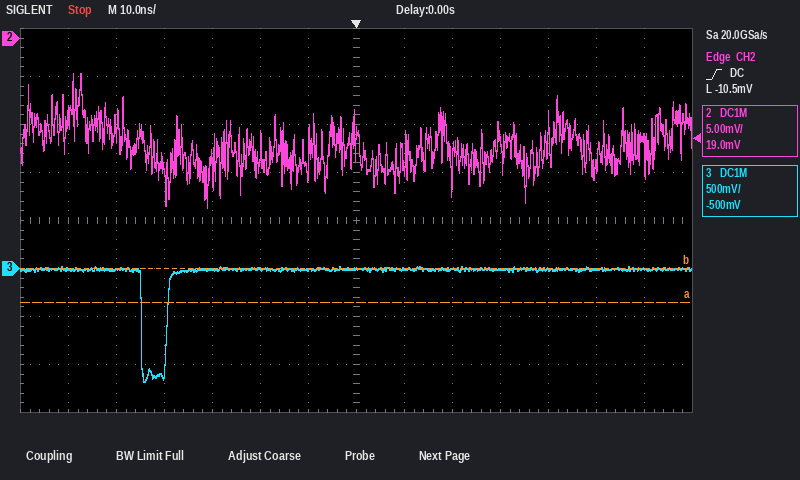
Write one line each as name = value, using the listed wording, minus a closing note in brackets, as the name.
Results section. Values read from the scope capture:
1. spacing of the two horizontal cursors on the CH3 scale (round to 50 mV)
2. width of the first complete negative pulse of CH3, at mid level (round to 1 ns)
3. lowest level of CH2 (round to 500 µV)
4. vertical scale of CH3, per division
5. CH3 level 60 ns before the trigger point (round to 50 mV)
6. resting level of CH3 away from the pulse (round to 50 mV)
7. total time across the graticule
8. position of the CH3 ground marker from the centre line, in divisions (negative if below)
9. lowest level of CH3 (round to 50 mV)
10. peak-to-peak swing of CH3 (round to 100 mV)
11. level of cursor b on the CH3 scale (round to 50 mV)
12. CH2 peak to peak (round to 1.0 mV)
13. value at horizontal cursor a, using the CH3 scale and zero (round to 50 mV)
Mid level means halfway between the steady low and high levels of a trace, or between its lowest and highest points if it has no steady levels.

spacing of the two horizontal cursors on the CH3 scale = 350 mV
width of the first complete negative pulse of CH3, at mid level = 5 ns
lowest level of CH2 = -17.5 mV
vertical scale of CH3, per division = 500 mV
CH3 level 60 ns before the trigger point = 0 mV
resting level of CH3 away from the pulse = 0 mV
total time across the graticule = 140 ns
position of the CH3 ground marker from the centre line, in divisions = -1.0 div
lowest level of CH3 = -1.20 V
peak-to-peak swing of CH3 = 1.20 V
level of cursor b on the CH3 scale = 0 mV
CH2 peak to peak = 14.0 mV
value at horizontal cursor a, using the CH3 scale and zero = -350 mV
